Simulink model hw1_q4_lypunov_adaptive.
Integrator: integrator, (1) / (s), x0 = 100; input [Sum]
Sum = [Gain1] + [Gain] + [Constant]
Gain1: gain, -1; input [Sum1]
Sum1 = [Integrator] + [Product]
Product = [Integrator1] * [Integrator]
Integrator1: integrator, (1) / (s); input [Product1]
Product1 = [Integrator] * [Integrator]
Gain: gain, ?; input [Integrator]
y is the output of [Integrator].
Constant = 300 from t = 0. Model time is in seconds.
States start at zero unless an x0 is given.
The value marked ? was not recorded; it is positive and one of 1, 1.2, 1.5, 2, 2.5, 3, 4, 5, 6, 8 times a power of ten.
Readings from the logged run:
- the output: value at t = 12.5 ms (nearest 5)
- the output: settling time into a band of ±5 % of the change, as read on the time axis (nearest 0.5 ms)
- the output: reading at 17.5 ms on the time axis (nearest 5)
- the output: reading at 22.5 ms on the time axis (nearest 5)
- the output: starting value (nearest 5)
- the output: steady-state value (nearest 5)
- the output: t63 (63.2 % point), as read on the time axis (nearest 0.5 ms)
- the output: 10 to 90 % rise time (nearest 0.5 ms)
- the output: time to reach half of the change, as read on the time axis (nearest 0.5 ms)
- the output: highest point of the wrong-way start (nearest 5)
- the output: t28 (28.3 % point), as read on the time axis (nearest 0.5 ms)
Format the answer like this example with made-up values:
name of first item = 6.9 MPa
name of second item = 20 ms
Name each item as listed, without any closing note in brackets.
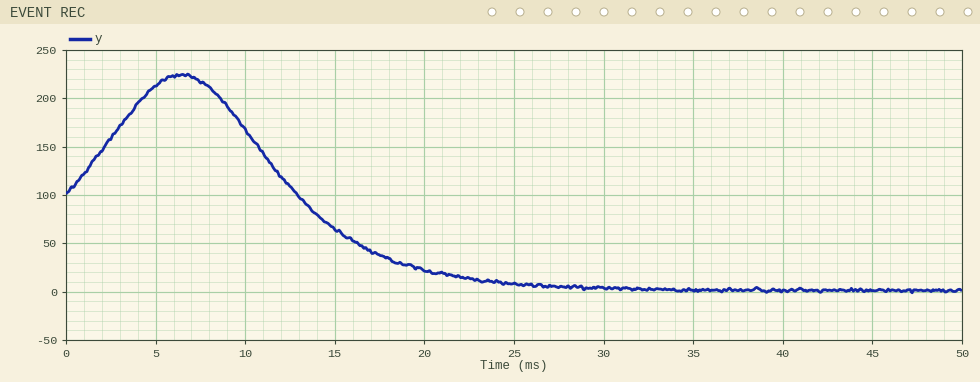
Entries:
the output: value at t = 12.5 ms = 110
the output: settling time into a band of ±5 % of the change, as read on the time axis = 26.5 ms
the output: reading at 17.5 ms on the time axis = 40
the output: reading at 22.5 ms on the time axis = 15
the output: starting value = 100
the output: steady-state value = 0
the output: t63 (63.2 % point), as read on the time axis = 17.5 ms
the output: 10 to 90 % rise time = 10.0 ms
the output: time to reach half of the change, as read on the time axis = 16.0 ms
the output: highest point of the wrong-way start = 225
the output: t28 (28.3 % point), as read on the time axis = 14.5 ms
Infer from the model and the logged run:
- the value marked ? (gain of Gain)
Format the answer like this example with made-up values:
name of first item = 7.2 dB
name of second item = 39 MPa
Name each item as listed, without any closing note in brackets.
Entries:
the value marked ? = 200
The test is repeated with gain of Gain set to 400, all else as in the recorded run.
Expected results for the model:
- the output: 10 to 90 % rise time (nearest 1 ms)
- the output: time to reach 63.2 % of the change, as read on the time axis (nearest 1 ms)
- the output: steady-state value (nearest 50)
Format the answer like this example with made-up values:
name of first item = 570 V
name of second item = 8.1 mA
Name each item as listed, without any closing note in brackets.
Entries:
the output: 10 to 90 % rise time = 5 ms
the output: time to reach 63.2 % of the change, as read on the time axis = 13 ms
the output: steady-state value = 0
